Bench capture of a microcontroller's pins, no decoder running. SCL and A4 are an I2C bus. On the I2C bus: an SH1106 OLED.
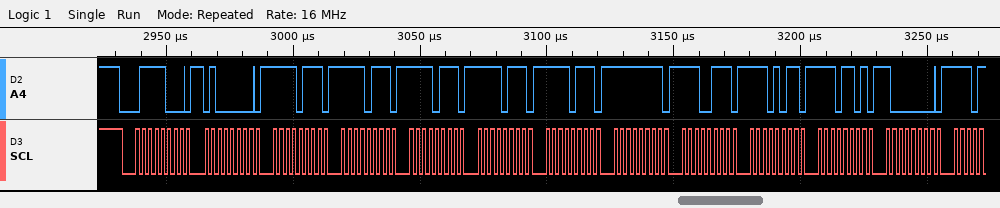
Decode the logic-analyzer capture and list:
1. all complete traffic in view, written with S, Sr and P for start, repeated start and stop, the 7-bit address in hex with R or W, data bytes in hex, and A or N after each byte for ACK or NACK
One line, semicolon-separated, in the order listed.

S 3CW A 40 A F7 A F7 A F7 A F7 A F7 A FF A E7 A EB A ED A 80 A
